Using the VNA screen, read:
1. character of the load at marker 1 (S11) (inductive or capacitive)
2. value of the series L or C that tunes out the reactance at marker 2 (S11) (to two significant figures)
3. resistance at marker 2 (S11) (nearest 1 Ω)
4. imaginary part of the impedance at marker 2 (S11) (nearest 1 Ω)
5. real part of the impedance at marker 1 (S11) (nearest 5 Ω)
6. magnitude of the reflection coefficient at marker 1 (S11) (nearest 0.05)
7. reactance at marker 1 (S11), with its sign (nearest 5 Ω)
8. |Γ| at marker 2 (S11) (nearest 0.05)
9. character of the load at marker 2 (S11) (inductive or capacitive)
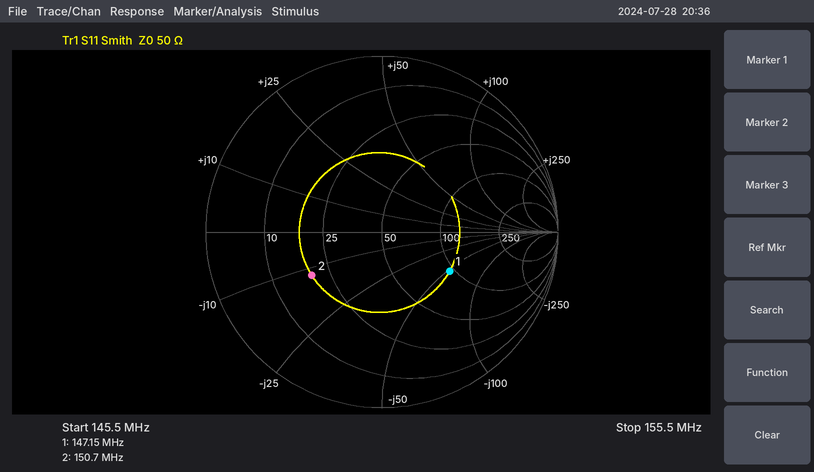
capacitive
13 nH
19 Ω
-12 Ω
95 Ω
0.45
-50 Ω
0.45
capacitive
